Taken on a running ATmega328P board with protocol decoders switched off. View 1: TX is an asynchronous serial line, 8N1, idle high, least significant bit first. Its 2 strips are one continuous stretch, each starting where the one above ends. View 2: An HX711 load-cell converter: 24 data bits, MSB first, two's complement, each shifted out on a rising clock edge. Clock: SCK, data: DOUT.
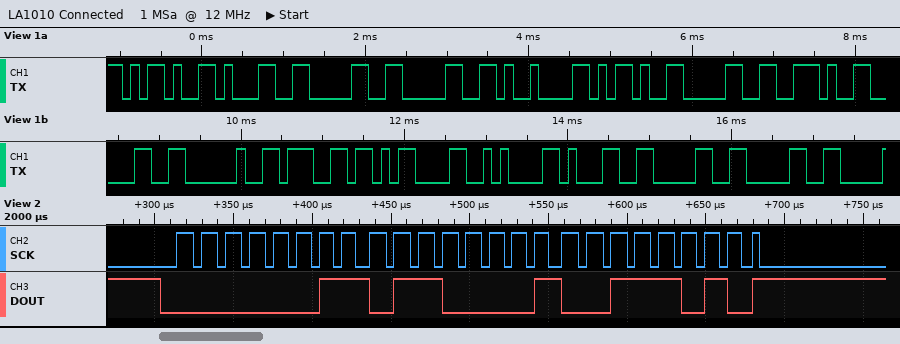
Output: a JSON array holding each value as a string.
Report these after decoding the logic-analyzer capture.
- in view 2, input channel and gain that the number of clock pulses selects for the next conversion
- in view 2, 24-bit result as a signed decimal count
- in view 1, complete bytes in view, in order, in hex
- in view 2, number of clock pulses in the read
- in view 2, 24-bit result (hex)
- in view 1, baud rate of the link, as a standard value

["channel A, gain 128", "221498", "2D 31 30 30 09 2D 30 2E 30 20 67 0D 0A 31 30 30", "25", "0x03613A", "9600 baud"]
